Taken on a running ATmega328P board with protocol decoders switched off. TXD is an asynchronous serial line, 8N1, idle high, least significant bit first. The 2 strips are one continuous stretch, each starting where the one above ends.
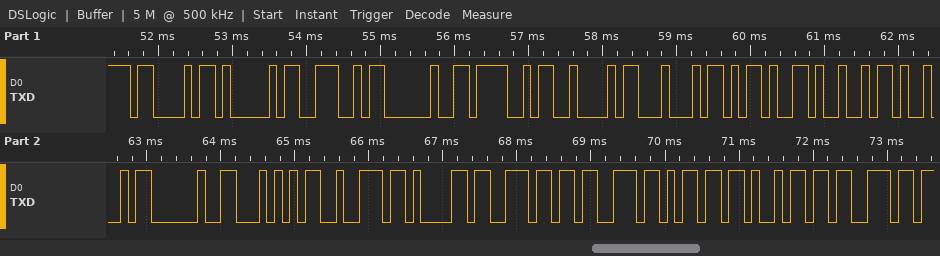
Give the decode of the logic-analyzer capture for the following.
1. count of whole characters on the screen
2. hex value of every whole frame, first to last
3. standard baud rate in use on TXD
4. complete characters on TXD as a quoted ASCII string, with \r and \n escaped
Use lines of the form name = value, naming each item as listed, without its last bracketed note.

count of whole characters on the screen = 19
hex value of every whole frame, first to last = 0x43 0x41 0x4E 0x20 0x4F 0x42 0x44 0x2D 0x49 0x49 0x20 0x54 0x72 0x61 0x6E 0x73 0x6D 0x69 0x73
standard baud rate in use on TXD = 9600 baud
complete characters on TXD as a quoted ASCII string, with \r and \n escaped = "CAN OBD-II Transmis"
